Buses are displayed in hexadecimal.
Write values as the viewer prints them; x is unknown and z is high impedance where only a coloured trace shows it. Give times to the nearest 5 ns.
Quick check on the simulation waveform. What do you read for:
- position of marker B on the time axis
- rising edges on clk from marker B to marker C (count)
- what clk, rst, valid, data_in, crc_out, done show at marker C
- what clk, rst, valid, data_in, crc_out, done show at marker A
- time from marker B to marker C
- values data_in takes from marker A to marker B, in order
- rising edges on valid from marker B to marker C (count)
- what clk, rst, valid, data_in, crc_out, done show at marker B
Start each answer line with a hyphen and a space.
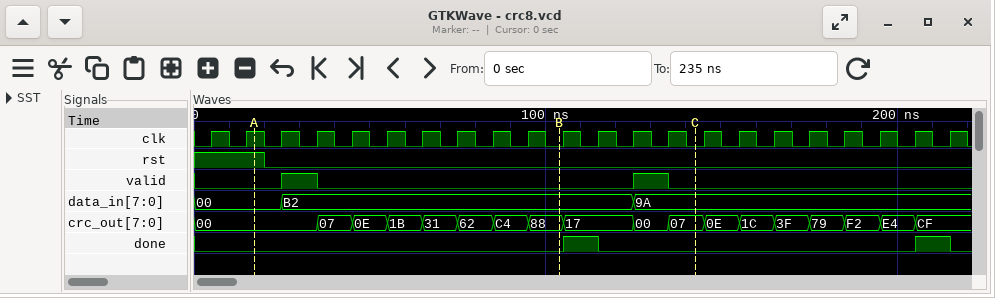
- 105 ns
- 4
- clk=0, rst=0, valid=0, data_in=9A, crc_out=07, done=0
- clk=1, rst=1, valid=0, data_in=00, crc_out=00, done=0
- 40 ns
- 00, B2
- 1
- clk=0, rst=0, valid=0, data_in=B2, crc_out=88, done=0
